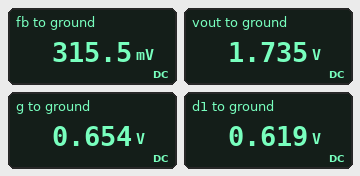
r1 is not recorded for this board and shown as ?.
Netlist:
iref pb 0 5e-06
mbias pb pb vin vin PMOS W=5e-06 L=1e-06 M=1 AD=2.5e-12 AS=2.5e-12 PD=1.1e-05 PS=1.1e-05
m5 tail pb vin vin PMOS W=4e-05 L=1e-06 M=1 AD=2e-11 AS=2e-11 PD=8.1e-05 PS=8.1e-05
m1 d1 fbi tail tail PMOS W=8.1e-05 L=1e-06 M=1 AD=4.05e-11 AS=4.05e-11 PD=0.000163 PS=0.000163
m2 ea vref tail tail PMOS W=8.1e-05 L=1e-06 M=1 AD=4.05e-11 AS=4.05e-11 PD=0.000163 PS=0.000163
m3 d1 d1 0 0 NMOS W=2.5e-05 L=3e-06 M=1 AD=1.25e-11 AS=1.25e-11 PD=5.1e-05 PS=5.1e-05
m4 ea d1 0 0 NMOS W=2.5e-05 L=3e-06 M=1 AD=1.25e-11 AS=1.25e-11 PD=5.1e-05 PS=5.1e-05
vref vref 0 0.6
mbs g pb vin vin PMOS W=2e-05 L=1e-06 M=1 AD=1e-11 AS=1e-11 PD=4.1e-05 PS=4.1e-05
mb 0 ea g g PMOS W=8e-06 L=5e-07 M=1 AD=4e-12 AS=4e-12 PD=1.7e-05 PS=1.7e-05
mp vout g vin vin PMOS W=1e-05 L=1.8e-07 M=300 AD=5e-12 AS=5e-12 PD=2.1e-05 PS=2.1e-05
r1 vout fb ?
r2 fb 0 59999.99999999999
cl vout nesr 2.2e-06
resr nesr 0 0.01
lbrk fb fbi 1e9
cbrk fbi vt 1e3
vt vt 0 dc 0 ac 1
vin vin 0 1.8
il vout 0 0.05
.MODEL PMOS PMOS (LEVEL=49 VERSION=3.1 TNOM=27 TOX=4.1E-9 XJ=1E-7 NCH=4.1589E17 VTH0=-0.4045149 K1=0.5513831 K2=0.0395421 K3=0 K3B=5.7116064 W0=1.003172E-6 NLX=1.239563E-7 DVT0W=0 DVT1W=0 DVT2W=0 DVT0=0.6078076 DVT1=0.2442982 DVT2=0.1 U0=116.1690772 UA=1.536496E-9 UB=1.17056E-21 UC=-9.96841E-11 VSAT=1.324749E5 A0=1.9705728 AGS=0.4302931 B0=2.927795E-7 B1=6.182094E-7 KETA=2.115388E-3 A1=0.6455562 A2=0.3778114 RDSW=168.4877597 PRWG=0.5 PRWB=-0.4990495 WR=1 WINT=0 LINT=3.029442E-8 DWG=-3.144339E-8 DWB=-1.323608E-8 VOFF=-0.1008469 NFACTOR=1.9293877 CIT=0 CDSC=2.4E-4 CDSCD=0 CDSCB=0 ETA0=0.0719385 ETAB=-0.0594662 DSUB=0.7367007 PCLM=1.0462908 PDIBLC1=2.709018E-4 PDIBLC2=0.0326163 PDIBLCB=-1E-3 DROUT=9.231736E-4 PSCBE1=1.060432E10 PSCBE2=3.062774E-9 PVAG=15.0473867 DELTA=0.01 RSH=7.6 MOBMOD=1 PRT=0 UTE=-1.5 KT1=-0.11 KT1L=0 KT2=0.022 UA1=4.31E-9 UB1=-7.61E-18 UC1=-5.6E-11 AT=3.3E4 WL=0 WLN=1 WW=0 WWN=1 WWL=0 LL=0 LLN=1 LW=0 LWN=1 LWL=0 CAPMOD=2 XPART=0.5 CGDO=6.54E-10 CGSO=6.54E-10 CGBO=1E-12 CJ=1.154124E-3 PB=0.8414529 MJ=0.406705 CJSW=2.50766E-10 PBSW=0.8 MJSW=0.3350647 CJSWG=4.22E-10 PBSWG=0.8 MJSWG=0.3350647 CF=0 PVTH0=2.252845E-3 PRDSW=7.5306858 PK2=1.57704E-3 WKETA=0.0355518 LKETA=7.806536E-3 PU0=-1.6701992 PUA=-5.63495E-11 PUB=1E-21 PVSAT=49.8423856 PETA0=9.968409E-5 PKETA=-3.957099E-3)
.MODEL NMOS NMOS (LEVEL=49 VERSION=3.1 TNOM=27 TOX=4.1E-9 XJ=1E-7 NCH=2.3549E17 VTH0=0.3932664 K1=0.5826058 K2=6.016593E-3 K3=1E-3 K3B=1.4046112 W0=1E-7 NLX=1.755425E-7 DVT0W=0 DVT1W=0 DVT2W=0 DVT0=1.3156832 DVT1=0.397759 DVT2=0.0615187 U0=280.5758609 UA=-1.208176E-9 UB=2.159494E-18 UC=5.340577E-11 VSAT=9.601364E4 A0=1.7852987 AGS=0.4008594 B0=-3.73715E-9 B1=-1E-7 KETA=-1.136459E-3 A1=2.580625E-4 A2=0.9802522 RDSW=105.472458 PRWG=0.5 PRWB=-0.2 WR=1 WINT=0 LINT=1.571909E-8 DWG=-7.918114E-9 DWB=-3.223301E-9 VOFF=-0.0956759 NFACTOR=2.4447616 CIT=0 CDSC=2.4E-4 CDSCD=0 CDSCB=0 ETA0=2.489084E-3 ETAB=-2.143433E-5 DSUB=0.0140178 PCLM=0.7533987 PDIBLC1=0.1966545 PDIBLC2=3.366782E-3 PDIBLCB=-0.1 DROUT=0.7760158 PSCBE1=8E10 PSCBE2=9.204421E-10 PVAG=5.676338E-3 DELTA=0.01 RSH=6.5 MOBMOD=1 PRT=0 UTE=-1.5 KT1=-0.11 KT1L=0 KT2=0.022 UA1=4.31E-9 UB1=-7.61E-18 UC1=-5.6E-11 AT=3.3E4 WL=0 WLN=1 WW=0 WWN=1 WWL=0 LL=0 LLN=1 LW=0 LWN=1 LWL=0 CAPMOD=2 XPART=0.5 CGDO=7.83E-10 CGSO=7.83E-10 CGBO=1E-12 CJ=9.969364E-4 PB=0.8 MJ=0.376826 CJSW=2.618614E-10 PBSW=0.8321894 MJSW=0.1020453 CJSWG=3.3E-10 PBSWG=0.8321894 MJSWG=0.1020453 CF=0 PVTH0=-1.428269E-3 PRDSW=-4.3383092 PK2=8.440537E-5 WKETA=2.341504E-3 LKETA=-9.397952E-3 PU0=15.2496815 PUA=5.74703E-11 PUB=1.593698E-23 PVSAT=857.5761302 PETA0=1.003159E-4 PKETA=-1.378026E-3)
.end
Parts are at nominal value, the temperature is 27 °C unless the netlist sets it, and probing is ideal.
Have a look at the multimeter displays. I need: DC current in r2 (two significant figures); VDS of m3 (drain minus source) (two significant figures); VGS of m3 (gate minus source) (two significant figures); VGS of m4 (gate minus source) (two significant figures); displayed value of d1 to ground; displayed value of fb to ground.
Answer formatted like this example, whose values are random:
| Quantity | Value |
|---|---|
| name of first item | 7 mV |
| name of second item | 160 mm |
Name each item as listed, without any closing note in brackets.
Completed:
| Quantity | Value |
|---|---|
| DC current in r2 | 5.3 µA |
| VDS of m3 (drain minus source) | 620 mV |
| VGS of m3 (gate minus source) | 620 mV |
| VGS of m4 (gate minus source) | 620 mV |
| displayed value of d1 to ground | 0.619 V |
| displayed value of fb to ground | 315.5 mV |
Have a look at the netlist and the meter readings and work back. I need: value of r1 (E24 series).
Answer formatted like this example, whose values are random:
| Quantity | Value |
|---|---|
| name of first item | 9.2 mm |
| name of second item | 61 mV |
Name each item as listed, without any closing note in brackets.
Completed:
| Quantity | Value |
|---|---|
| value of r1 | 270 kΩ |
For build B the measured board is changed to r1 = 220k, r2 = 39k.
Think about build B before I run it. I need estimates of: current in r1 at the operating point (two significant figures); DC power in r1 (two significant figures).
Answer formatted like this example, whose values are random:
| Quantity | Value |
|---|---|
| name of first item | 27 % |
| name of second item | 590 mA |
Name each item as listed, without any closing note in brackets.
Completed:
| Quantity | Value |
|---|---|
| current in r1 at the operating point | 6.7 µA |
| DC power in r1 | 9.9 µW |
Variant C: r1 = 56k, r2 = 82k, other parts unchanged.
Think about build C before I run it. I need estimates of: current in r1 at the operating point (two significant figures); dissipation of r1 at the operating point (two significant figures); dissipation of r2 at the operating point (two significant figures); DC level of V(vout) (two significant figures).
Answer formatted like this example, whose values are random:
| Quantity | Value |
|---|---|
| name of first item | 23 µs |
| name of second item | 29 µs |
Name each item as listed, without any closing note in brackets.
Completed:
| Quantity | Value |
|---|---|
| current in r1 at the operating point | 7.3 µA |
| dissipation of r1 at the operating point | 3.0 µW |
| dissipation of r2 at the operating point | 4.4 µW |
| DC level of V(vout) | 1.0 V |
